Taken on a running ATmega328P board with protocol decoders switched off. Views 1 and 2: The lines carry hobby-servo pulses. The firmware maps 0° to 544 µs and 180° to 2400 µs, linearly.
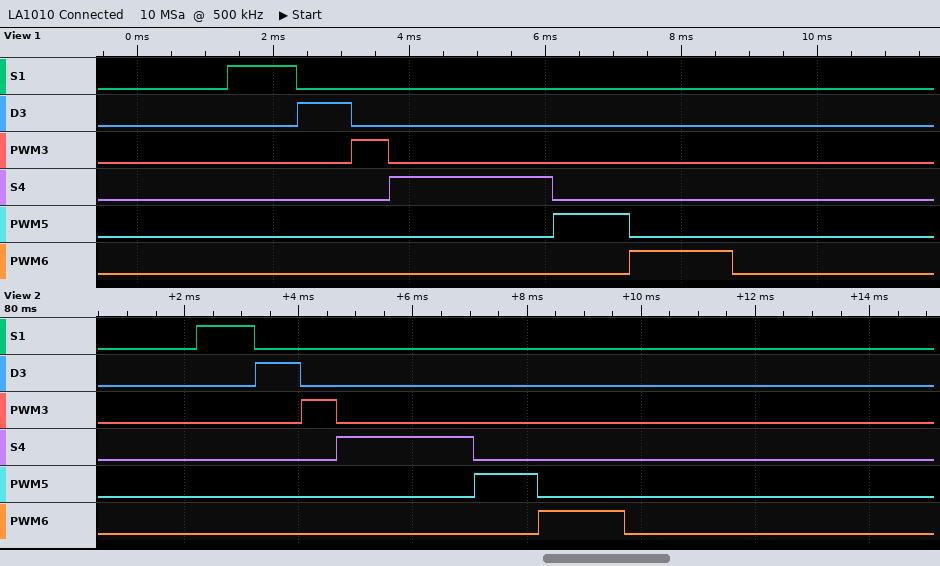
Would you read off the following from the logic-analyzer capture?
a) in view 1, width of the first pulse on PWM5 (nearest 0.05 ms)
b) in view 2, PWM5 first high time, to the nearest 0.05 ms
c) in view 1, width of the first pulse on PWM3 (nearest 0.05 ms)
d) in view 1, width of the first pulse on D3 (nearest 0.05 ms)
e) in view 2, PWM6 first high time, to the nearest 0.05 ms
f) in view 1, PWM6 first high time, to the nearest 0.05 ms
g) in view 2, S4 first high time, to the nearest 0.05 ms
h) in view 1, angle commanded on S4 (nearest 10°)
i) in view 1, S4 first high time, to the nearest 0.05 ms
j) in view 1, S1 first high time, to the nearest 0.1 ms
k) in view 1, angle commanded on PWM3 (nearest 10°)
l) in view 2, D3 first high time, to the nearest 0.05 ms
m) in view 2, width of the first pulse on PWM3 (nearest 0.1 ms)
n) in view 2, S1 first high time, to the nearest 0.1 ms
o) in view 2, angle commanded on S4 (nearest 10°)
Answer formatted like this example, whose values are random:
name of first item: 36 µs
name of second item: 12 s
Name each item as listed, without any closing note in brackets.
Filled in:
in view 1, width of the first pulse on PWM5: 1.10 ms
in view 2, PWM5 first high time, to the nearest 0.05 ms: 1.10 ms
in view 1, width of the first pulse on PWM3: 0.55 ms
in view 1, width of the first pulse on D3: 0.80 ms
in view 2, PWM6 first high time, to the nearest 0.05 ms: 1.50 ms
in view 1, PWM6 first high time, to the nearest 0.05 ms: 1.50 ms
in view 2, S4 first high time, to the nearest 0.05 ms: 2.40 ms
in view 1, angle commanded on S4: 180°
in view 1, S4 first high time, to the nearest 0.05 ms: 2.40 ms
in view 1, S1 first high time, to the nearest 0.1 ms: 1.0 ms
in view 1, angle commanded on PWM3: 0°
in view 2, D3 first high time, to the nearest 0.05 ms: 0.80 ms
in view 2, width of the first pulse on PWM3: 0.6 ms
in view 2, S1 first high time, to the nearest 0.1 ms: 1.0 ms
in view 2, angle commanded on S4: 180°
